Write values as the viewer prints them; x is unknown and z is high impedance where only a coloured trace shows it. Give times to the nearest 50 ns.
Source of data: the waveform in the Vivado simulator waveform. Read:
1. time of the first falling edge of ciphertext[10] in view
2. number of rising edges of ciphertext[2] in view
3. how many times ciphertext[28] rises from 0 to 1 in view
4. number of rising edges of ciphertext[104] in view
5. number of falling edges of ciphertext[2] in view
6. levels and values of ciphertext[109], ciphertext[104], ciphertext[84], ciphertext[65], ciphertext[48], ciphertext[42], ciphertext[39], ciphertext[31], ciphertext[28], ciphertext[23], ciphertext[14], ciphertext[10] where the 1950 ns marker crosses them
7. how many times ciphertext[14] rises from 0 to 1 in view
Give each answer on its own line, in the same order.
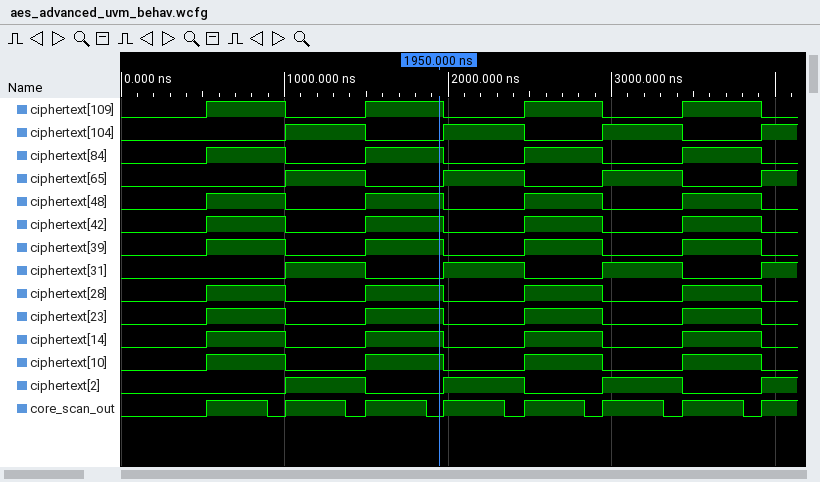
1000 ns
4
4
4
3
ciphertext[109]=1, ciphertext[104]=0, ciphertext[84]=1, ciphertext[65]=0, ciphertext[48]=1, ciphertext[42]=1, ciphertext[39]=1, ciphertext[31]=0, ciphertext[28]=1, ciphertext[23]=1, ciphertext[14]=1, ciphertext[10]=1
4
